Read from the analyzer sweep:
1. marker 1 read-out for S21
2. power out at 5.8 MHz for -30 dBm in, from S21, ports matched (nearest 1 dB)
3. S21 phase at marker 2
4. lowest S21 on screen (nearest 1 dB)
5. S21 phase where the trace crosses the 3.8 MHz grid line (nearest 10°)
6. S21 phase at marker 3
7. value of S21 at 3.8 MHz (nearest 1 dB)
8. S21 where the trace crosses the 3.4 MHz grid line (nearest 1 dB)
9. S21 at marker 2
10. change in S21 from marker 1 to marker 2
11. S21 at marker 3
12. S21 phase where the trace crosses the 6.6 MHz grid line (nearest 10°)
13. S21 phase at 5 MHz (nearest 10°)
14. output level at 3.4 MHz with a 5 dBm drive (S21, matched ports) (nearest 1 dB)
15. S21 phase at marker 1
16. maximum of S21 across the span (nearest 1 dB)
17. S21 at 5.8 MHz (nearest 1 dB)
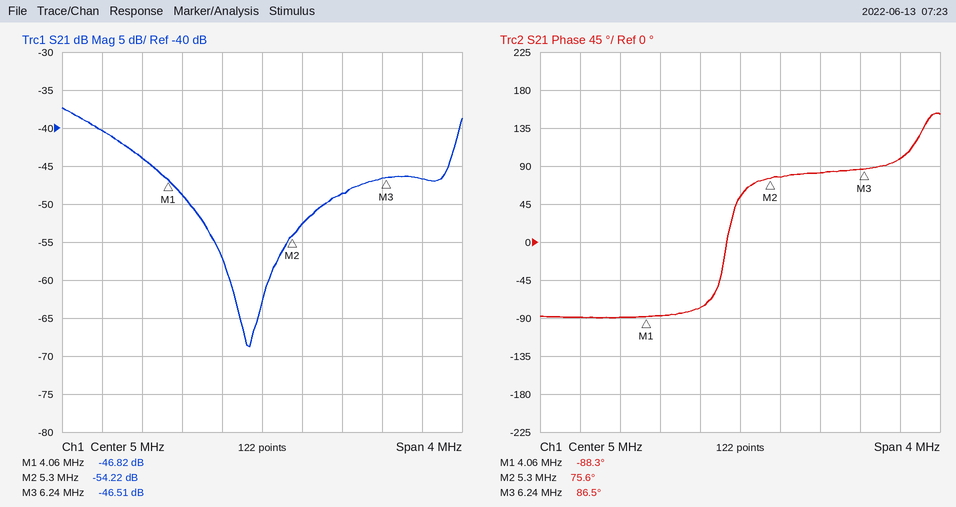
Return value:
-46.82 dB
-79 dBm
75.6°
-69 dB
-90°
86.5°
-44 dB
-40 dB
-54.22 dB
-7.40 dB
-46.51 dB
100°
50°
-35 dBm
-88.3°
-37 dB
-49 dB
